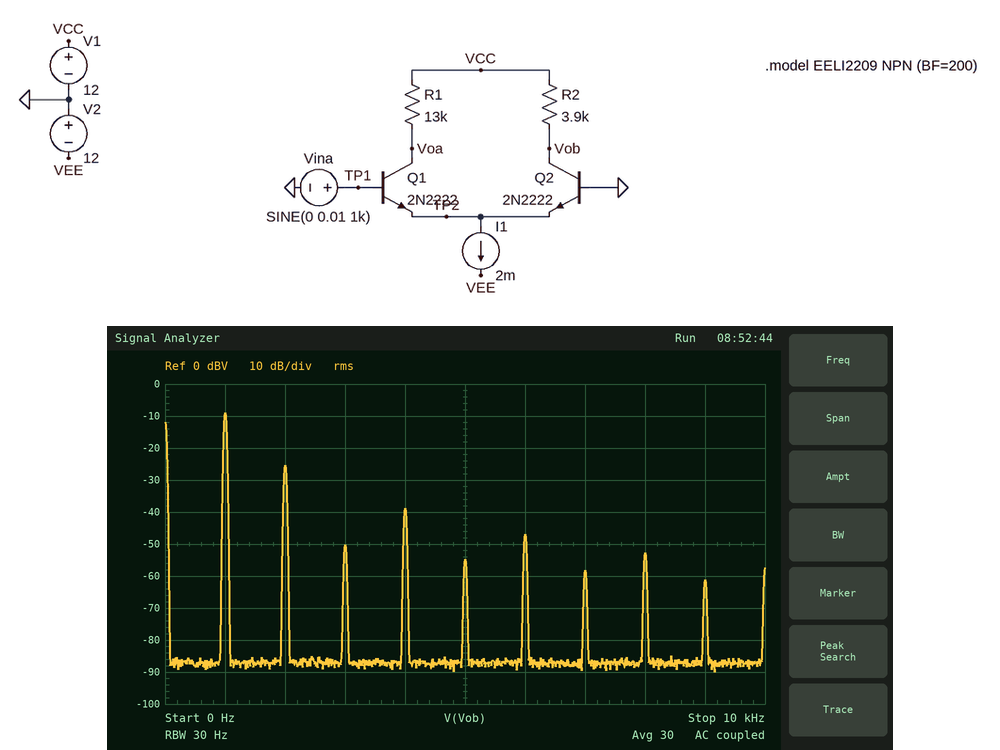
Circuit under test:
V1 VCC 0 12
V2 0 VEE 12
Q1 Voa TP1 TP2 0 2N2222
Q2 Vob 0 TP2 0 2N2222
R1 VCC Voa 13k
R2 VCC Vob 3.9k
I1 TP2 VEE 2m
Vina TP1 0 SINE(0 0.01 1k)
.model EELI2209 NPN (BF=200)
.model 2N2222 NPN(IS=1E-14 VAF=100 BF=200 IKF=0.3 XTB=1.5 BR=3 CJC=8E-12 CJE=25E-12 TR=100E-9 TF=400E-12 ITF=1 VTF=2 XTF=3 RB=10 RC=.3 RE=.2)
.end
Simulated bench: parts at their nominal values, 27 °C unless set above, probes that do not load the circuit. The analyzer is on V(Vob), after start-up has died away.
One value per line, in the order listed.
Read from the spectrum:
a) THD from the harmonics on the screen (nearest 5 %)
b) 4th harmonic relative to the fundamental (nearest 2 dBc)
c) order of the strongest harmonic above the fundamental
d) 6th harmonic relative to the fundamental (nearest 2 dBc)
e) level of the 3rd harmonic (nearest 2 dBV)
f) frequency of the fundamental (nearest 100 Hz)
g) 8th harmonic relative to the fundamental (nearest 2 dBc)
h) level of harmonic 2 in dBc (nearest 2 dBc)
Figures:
15 %
-30 dBc
2
-38 dBc
-50 dBV
1.0 kHz
-44 dBc
-16 dBc
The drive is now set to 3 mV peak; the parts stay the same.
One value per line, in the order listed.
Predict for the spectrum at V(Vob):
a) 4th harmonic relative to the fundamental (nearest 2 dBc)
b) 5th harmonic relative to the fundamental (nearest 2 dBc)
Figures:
-34 dBc
-40 dBc
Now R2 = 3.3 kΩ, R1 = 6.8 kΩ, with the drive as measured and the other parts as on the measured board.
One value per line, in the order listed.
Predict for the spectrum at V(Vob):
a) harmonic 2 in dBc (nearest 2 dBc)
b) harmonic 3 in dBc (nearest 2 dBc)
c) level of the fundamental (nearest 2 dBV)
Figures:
-58 dBc
-52 dBc
-8 dBV
